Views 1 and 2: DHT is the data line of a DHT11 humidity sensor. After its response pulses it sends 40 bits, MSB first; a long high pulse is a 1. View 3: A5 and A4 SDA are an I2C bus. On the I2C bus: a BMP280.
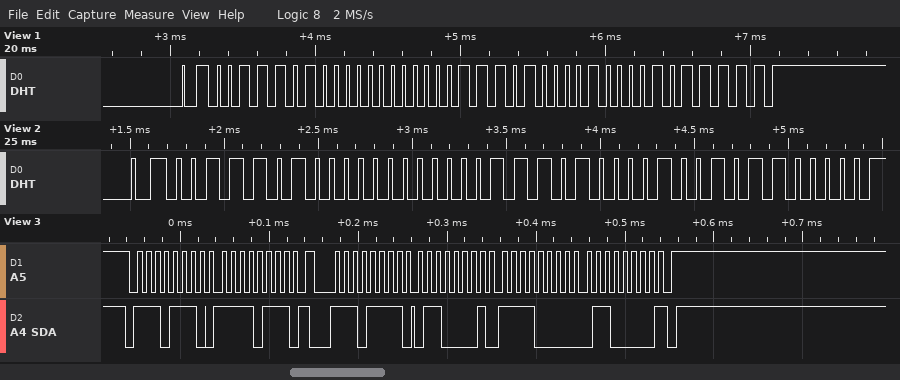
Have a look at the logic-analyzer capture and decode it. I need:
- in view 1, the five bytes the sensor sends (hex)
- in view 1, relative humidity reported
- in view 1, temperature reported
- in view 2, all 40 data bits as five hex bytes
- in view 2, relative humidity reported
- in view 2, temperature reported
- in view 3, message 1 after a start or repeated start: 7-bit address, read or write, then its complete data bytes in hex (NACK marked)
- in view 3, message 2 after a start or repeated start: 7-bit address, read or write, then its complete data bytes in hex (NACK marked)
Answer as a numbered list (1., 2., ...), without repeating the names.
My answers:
1. 3A 00 1D 08 5F
2. 58 %
3. 29.8 °C
4. 3A 00 1D 09 60
5. 58 %
6. 29.9 °C
7. 0x77 write: F7
8. 0x77 read: 61 F0 60 NACK
